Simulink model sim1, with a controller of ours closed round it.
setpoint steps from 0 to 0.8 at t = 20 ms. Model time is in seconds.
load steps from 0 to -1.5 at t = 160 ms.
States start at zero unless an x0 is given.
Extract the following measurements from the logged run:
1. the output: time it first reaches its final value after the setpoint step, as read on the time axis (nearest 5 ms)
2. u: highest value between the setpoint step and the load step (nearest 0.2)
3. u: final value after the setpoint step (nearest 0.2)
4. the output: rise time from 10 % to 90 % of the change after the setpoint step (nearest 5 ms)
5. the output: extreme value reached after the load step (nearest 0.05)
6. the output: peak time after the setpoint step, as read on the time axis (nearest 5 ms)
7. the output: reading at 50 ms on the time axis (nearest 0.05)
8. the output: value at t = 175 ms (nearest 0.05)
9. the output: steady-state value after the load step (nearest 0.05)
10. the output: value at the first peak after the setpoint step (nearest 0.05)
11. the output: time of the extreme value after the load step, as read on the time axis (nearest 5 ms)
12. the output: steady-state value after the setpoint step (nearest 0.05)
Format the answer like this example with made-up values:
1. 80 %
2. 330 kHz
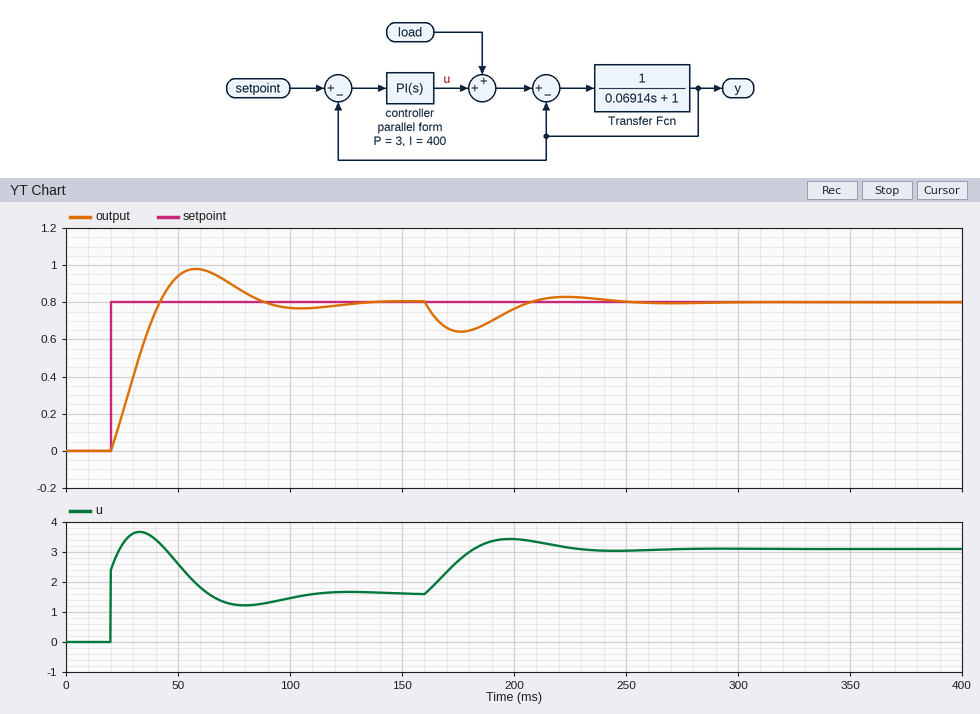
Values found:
1. 40 ms
2. 3.6
3. 1.6
4. 15 ms
5. 0.65
6. 60 ms
7. 0.95
8. 0.65
9. 0.80
10. 1.00
11. 175 ms
12. 0.80
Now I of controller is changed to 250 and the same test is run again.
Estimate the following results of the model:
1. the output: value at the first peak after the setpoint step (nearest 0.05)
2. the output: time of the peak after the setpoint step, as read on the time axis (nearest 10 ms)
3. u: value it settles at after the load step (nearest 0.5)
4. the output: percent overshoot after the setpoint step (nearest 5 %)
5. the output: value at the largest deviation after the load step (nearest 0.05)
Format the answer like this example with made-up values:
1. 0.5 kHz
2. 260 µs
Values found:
1. 0.90
2. 70 ms
3. 3.0
4. 15 %
5. 0.60
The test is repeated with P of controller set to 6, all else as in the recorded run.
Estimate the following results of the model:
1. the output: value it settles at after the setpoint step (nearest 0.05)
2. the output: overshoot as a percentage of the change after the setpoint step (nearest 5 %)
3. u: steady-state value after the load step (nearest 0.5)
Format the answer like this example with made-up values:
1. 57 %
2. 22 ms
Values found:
1. 0.80
2. 10 %
3. 3.0
